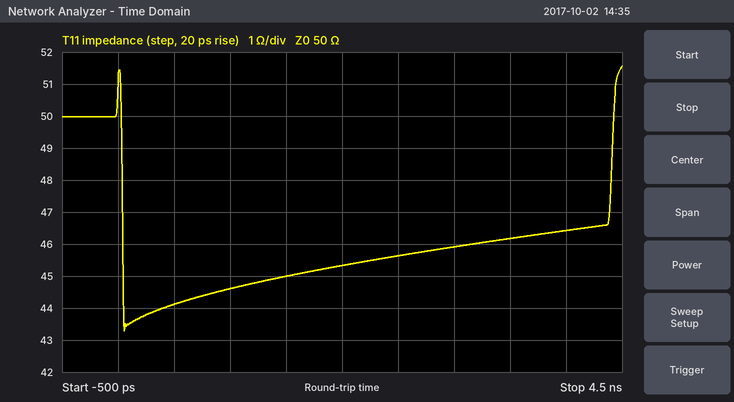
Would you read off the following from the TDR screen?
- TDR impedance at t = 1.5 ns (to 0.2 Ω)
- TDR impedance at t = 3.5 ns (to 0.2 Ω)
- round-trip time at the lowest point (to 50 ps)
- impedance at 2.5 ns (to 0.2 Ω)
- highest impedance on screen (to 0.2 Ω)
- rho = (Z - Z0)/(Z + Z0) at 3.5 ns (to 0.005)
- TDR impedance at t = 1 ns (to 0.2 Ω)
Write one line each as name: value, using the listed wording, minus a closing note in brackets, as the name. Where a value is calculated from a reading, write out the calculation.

TDR impedance at t = 1.5 ns: 45.0 Ω
TDR impedance at t = 3.5 ns: 46.2 Ω
round-trip time at the lowest point: 50 ps
impedance at 2.5 ns: 45.6 Ω
highest impedance on screen: 51.6 Ω
rho = (Z - Z0)/(Z + Z0) at 3.5 ns: (46.2 − 50)/(46.2 + 50) ≈ -0.040
TDR impedance at t = 1 ns: 44.6 Ω
